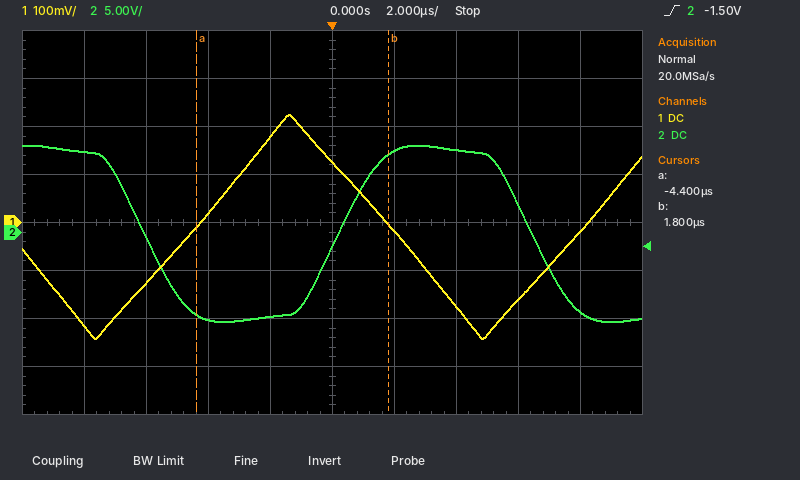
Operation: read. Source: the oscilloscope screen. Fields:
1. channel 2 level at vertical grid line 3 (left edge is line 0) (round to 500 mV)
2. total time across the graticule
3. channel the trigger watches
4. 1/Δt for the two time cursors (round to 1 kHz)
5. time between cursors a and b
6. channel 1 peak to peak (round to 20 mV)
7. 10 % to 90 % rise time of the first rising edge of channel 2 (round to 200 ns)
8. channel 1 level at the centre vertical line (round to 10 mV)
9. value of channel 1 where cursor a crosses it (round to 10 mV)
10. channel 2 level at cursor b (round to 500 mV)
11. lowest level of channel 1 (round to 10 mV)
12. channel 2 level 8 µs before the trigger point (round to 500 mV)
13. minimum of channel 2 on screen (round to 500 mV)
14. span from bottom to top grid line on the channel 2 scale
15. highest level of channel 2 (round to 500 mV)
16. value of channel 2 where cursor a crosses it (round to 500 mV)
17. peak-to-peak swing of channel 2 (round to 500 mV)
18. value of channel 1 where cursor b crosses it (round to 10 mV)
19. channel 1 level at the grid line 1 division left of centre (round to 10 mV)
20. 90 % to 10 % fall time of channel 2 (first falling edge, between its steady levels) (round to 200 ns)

-9.0 V
20 µs
channel 2
161 kHz
6.2 µs
460 mV
2.4 µs
130 mV
-10 mV
8.0 V
-240 mV
8.5 V
-9.5 V
40 V
9.0 V
-8.5 V
18.5 V
0 mV
180 mV
2.4 µs
